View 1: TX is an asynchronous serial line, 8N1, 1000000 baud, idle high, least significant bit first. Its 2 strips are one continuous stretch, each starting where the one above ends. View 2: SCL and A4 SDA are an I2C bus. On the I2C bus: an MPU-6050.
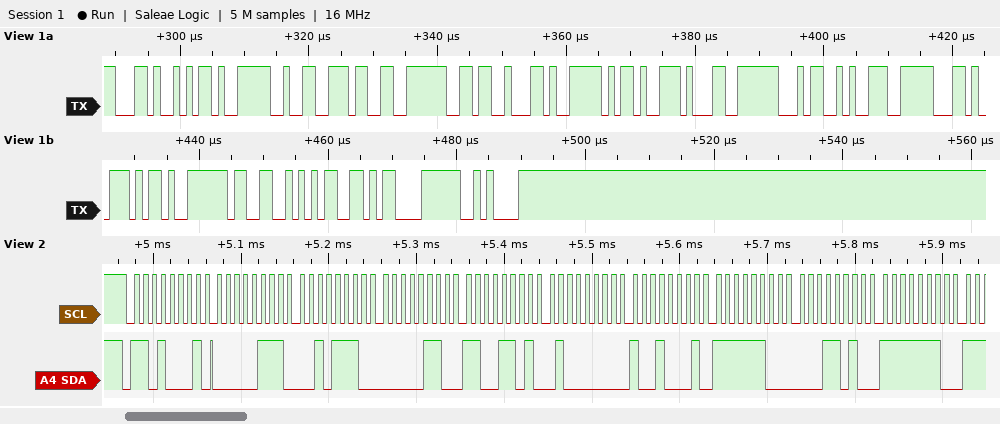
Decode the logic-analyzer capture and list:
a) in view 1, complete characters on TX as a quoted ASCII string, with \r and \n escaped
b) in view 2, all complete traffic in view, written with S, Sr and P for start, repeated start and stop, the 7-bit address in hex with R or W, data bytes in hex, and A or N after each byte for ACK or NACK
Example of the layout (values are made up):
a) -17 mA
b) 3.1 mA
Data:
a) ",-236,-149,-35\r\n"
b) S 68R A 07 A 2E A 06 A CD A 40 A 91 A FC A 1A A FE A
